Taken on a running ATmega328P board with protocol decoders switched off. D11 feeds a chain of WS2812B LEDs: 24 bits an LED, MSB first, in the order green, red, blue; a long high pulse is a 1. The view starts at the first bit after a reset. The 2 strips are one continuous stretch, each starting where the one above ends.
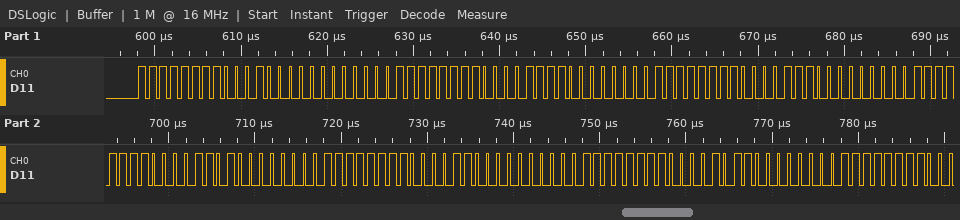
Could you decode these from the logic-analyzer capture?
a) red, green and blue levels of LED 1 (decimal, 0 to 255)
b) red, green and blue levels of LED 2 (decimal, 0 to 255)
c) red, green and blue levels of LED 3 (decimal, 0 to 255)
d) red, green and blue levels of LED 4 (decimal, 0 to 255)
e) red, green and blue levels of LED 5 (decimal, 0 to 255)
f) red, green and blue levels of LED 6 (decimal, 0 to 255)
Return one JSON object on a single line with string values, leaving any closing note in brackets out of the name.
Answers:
{"red, green and blue levels of LED 1": "16, 255, 0", "red, green and blue levels of LED 2": "15, 255, 0", "red, green and blue levels of LED 3": "14, 255, 0", "red, green and blue levels of LED 4": "13, 255, 0", "red, green and blue levels of LED 5": "12, 255, 0", "red, green and blue levels of LED 6": "11, 255, 0"}
